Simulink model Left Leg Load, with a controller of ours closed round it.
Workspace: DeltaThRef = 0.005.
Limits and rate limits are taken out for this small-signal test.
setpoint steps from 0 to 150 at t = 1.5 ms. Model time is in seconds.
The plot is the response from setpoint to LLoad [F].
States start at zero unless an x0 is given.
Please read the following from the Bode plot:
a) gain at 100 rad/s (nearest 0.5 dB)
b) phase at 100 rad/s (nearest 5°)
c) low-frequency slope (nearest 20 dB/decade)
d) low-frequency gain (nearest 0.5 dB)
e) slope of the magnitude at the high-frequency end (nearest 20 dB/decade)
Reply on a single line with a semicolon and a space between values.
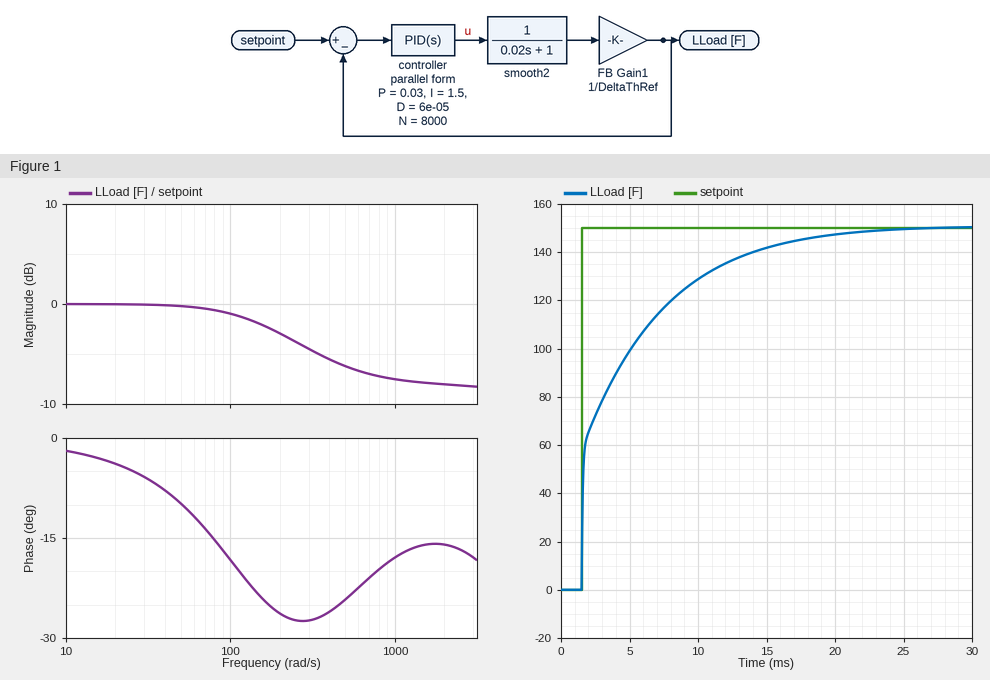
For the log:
-1.0 dB; -20°; 0 dB/decade; 0.0 dB; 0 dB/decade
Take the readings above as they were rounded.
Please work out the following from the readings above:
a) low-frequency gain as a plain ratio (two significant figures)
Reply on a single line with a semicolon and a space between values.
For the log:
1.0
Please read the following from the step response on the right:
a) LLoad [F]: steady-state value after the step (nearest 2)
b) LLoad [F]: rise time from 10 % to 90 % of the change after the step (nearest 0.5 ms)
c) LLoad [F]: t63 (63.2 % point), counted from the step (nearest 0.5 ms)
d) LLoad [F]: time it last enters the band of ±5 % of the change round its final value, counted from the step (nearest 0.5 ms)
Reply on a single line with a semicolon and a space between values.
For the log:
150; 10.5 ms; 3.0 ms; 14.0 ms
